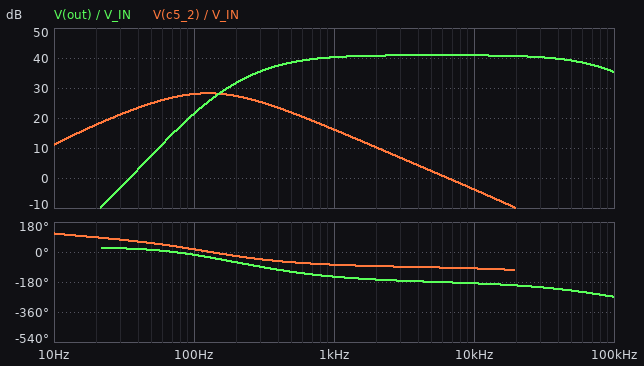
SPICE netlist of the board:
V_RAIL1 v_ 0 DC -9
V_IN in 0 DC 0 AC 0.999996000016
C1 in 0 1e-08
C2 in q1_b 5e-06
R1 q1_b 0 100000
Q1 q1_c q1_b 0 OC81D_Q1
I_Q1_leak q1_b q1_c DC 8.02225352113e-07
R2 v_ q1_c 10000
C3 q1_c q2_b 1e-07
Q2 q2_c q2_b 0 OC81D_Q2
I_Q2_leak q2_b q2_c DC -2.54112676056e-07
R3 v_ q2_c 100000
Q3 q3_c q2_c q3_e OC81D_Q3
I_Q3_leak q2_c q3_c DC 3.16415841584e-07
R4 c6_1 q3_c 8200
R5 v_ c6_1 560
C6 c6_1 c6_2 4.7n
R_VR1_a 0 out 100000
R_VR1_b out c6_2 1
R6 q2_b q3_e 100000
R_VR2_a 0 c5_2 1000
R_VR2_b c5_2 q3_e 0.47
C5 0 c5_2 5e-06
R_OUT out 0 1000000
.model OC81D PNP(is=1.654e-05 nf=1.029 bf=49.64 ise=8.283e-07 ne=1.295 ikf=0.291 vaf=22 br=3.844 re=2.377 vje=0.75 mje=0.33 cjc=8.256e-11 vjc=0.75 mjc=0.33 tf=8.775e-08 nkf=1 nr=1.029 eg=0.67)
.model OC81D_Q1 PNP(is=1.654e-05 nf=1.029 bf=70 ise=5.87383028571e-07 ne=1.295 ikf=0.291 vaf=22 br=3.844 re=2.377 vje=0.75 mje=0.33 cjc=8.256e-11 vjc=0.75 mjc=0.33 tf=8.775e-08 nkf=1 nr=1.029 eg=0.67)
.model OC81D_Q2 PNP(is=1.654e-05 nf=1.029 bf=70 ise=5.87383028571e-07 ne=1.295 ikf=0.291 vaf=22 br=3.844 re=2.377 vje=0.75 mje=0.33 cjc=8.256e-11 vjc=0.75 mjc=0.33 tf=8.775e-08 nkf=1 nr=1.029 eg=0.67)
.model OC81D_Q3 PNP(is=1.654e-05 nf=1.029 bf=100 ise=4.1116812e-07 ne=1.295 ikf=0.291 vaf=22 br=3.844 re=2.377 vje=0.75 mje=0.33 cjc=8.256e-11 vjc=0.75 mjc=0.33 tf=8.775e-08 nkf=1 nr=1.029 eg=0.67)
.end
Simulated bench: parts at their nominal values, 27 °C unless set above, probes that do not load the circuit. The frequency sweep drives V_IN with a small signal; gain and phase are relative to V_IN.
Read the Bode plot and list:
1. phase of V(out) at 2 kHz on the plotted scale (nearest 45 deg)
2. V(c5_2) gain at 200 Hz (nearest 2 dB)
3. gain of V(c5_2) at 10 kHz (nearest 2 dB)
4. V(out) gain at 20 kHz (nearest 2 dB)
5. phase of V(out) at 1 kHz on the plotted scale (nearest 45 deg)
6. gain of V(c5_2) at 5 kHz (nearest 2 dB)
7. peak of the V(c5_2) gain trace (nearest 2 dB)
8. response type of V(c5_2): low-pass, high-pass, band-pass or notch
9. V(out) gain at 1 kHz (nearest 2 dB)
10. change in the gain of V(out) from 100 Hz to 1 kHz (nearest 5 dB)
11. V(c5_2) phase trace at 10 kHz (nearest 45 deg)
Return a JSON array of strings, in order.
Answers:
["-180 deg", "28 dB", "-4 dB", "40 dB", "-135 deg", "2 dB", "28 dB", "band-pass", "40 dB", "20 dB", "-90 deg"]
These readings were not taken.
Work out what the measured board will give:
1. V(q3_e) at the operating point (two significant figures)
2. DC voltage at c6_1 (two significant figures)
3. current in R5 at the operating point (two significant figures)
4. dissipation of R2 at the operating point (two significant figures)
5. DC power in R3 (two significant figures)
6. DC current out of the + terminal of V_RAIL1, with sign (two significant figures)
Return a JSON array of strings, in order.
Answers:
["-56 mV", "-9.0 V", "60 µA", "380 µW", "800 µW", "-340 µA"]
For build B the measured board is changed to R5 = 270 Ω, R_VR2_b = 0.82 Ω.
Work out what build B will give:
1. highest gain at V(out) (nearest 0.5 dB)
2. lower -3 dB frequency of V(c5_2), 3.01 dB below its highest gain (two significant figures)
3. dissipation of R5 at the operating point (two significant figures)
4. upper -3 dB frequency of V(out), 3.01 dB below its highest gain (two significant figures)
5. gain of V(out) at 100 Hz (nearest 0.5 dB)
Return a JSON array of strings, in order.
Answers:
["34.5 dB", "52 Hz", "970 nW", "68 kHz", "15.0 dB"]
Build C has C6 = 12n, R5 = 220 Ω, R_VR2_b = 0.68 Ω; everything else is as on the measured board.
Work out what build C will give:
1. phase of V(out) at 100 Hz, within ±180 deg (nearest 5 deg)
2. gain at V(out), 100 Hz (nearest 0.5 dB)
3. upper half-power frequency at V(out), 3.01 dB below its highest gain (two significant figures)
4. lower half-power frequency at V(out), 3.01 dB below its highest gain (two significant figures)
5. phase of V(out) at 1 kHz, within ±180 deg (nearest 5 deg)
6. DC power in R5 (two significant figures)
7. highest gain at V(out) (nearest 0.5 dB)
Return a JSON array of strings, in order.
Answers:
["-35 deg", "20.0 dB", "68 kHz", "260 Hz", "-160 deg", "790 nW", "33.0 dB"]
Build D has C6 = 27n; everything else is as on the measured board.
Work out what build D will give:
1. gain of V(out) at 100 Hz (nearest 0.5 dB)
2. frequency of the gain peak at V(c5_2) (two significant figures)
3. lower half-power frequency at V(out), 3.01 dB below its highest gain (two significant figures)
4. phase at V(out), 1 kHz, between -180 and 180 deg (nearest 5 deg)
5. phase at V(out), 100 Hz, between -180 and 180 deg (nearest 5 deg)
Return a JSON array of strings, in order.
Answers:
["31.5 dB", "130 Hz", "210 Hz", "-165 deg", "-60 deg"]
